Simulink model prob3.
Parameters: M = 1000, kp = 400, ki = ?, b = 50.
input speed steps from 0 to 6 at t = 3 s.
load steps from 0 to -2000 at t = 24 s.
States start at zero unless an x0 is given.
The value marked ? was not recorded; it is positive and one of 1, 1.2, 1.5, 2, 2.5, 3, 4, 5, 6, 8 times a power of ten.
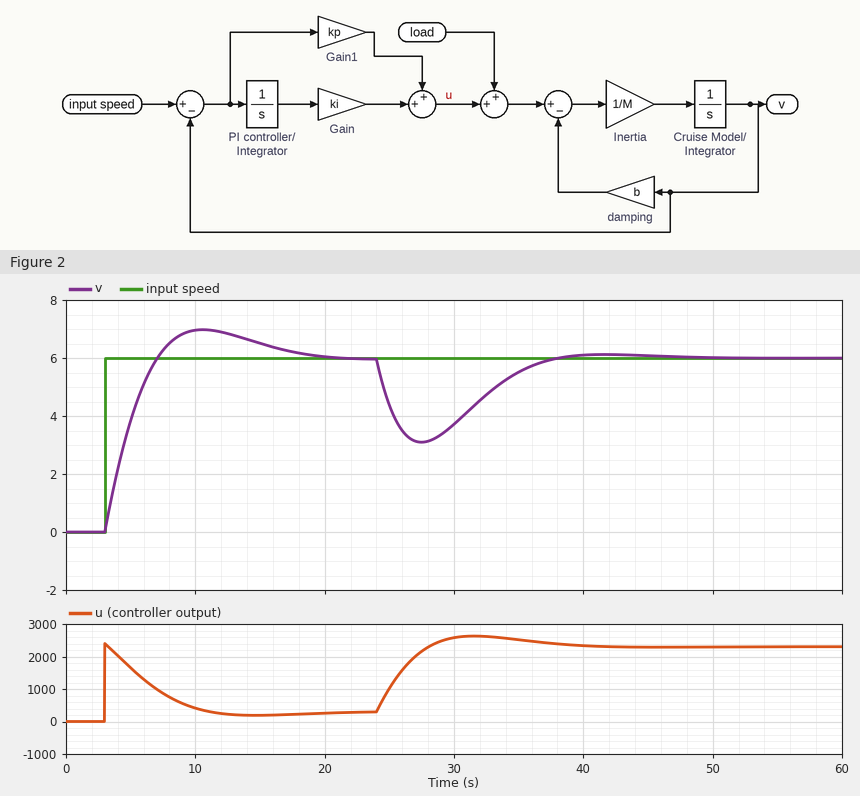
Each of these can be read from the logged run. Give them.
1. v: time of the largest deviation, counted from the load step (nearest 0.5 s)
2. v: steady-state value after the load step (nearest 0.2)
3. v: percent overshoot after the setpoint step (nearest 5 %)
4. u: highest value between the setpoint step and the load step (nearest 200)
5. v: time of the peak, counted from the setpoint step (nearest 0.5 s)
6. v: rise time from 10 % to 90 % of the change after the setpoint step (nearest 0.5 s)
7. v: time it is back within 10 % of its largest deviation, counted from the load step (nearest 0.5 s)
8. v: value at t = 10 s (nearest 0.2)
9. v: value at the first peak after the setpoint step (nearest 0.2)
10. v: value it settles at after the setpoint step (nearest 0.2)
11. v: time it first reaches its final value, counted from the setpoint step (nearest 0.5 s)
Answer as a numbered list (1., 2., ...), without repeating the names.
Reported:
1. 3.5 s
2. 6.0
3. 15 %
4. 2400
5. 7.5 s
6. 3.0 s
7. 12.0 s
8. 7.0
9. 7.0
10. 6.0
11. 4.0 s
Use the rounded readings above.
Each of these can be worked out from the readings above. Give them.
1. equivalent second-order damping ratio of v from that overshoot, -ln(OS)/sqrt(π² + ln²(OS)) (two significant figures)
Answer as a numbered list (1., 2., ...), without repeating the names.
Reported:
1. 0.52
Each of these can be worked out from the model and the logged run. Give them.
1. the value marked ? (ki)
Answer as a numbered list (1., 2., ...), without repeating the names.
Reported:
1. 100
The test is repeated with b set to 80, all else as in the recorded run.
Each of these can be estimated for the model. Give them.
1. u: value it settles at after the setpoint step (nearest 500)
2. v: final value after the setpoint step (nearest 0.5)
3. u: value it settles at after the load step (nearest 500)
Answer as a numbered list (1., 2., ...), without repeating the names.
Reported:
1. 500
2. 6.0
3. 2500
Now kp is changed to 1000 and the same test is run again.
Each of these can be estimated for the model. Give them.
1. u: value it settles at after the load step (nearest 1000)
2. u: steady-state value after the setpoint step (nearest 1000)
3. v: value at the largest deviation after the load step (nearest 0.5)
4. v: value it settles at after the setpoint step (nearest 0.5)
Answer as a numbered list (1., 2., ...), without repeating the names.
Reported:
1. 2000
2. 0
3. 4.5
4. 6.0
